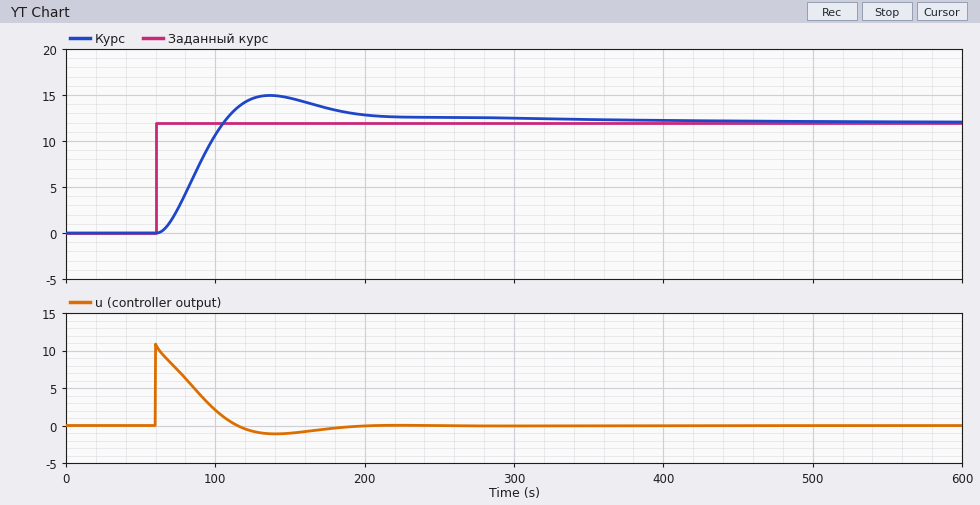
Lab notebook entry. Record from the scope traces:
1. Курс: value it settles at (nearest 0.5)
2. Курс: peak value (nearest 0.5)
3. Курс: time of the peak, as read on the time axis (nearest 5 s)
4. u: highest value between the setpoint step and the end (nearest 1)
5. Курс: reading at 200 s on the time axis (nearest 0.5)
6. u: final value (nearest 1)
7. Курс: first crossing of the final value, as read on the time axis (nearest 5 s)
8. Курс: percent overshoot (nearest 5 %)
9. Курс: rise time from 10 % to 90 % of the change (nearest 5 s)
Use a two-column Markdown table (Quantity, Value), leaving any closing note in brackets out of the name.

| Quantity | Value |
|---|---|
| Курс: value it settles at | 12.0 |
| Курс: peak value | 15.0 |
| Курс: time of the peak, as read on the time axis | 135 s |
| u: highest value between the setpoint step and the end | 11 |
| Курс: reading at 200 s on the time axis | 13.0 |
| u: final value | 0 |
| Курс: first crossing of the final value, as read on the time axis | 105 s |
| Курс: percent overshoot | 25 % |
| Курс: rise time from 10 % to 90 % of the change | 30 s |
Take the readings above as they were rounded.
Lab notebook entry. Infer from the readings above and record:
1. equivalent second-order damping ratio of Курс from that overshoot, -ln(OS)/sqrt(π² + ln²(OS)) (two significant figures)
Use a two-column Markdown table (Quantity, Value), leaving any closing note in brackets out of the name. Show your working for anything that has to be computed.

| Quantity | Value |
|---|---|
| equivalent second-order damping ratio of Курс from that overshoot, -ln(OS)/sqrt(π² + ln²(OS)) | ln(0.25) = -1.386; 1.386 / sqrt(9.870 + 1.922) = 0.40 |
